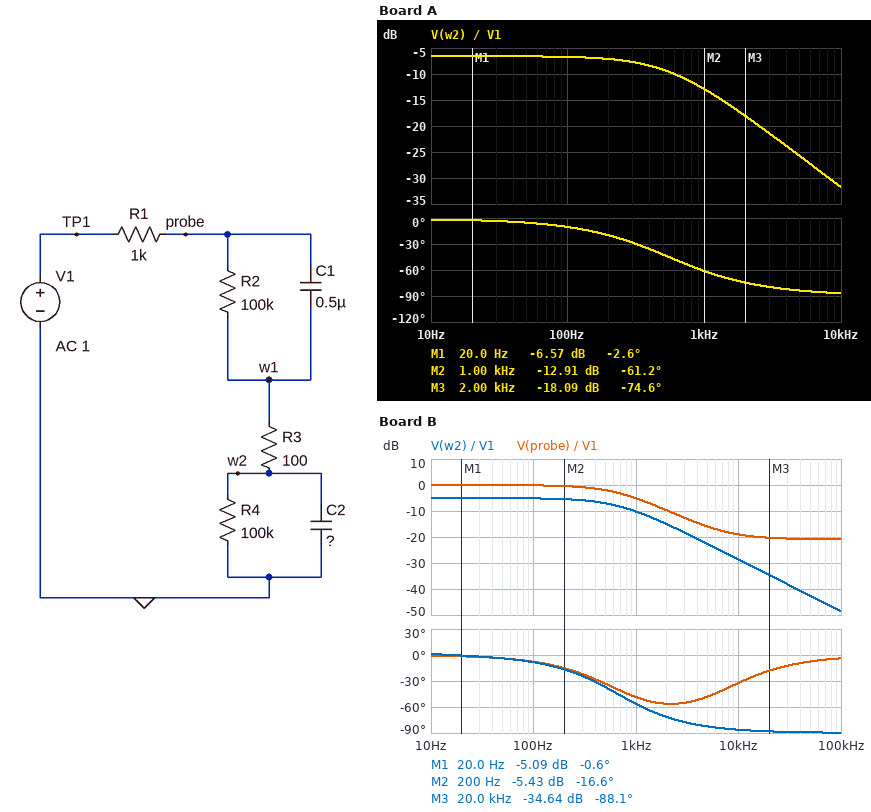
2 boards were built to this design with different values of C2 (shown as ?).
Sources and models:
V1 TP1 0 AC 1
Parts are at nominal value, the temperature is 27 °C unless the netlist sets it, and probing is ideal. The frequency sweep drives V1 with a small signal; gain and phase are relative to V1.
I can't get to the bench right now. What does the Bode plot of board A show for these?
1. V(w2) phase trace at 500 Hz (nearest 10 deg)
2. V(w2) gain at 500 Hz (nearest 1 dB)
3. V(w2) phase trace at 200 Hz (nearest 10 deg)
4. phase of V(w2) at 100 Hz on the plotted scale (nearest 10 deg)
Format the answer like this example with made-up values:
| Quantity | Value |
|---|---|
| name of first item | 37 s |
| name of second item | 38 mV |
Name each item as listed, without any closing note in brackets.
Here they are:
| Quantity | Value |
|---|---|
| V(w2) phase trace at 500 Hz | -40 deg |
| V(w2) gain at 500 Hz | -9 dB |
| V(w2) phase trace at 200 Hz | -20 deg |
| phase of V(w2) at 100 Hz on the plotted scale | -10 deg |
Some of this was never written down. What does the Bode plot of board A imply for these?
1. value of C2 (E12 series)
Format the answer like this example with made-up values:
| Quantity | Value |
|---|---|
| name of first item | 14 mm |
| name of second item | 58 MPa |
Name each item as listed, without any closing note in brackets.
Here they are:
| Quantity | Value |
|---|---|
| value of C2 | 560 nF |
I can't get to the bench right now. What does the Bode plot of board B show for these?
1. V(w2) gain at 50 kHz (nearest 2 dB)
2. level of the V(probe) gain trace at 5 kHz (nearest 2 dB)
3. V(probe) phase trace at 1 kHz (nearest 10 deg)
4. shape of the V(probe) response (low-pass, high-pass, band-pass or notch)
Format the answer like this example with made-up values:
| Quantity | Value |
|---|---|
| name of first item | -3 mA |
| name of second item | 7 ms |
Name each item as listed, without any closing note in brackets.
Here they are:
| Quantity | Value |
|---|---|
| V(w2) gain at 50 kHz | -42 dB |
| level of the V(probe) gain trace at 5 kHz | -16 dB |
| V(probe) phase trace at 1 kHz | -50 deg |
| shape of the V(probe) response | low-pass |
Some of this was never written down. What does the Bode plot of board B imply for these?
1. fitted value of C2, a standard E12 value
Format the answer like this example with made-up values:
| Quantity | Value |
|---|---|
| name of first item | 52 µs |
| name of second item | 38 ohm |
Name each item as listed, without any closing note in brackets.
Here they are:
| Quantity | Value |
|---|---|
| fitted value of C2, a standard E12 value | 390 nF |
